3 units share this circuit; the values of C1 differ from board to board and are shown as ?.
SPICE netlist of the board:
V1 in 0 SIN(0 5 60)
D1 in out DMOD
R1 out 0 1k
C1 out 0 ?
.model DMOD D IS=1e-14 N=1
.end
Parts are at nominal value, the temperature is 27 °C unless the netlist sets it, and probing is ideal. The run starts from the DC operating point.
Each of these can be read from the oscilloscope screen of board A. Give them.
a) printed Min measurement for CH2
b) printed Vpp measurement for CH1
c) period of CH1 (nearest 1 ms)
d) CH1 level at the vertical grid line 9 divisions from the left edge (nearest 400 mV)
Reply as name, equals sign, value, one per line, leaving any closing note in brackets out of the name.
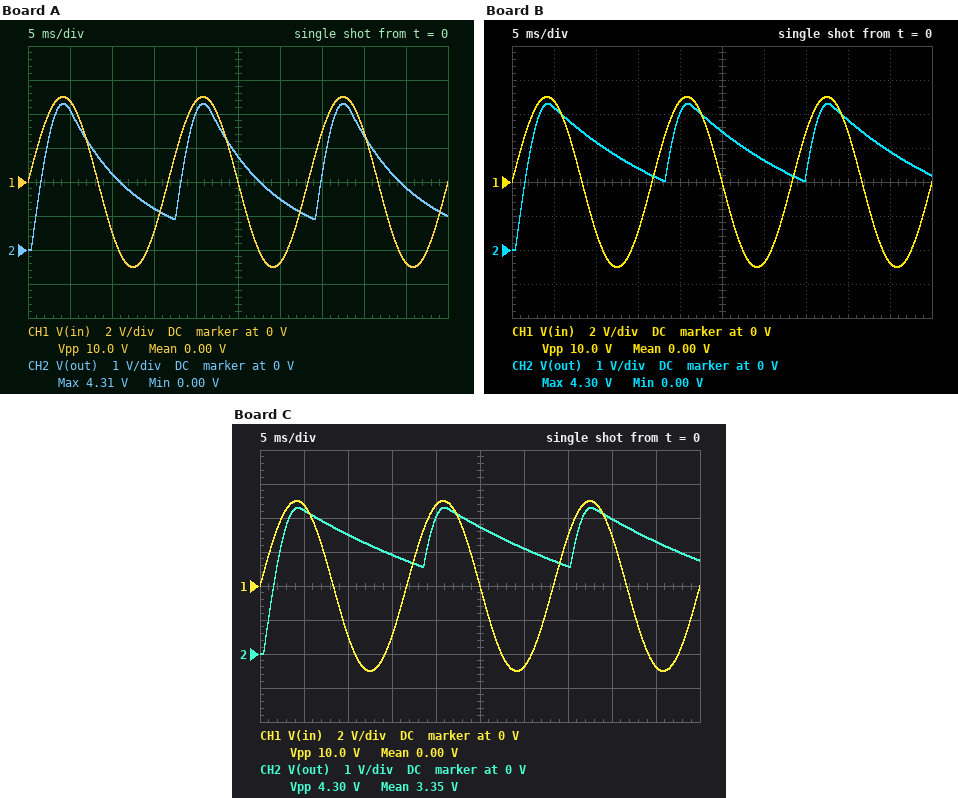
printed Min measurement for CH2 = 0.00 V
printed Vpp measurement for CH1 = 10.0 V
period of CH1 = 17 ms
CH1 level at the vertical grid line 9 divisions from the left edge = -4.8 V
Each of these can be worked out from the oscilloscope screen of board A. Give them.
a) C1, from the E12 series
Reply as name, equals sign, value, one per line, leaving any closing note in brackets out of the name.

C1, from the E12 series = 8.2 µF
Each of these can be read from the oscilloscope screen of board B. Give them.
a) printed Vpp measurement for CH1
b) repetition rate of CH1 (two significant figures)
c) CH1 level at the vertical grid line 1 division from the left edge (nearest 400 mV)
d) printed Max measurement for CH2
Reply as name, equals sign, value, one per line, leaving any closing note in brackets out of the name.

printed Vpp measurement for CH1 = 10.0 V
repetition rate of CH1 = 60 Hz
CH1 level at the vertical grid line 1 division from the left edge = 4.8 V
printed Max measurement for CH2 = 4.30 V
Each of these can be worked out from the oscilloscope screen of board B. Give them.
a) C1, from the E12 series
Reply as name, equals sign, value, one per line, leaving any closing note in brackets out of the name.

C1, from the E12 series = 18 µF
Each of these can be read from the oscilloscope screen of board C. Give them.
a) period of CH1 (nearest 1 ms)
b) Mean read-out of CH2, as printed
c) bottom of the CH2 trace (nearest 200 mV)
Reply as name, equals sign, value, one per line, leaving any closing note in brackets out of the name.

period of CH1 = 17 ms
Mean read-out of CH2, as printed = 3.35 V
bottom of the CH2 trace = 0 V
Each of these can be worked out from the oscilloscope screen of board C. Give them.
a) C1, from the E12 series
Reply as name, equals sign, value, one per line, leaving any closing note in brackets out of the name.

C1, from the E12 series = 27 µF
